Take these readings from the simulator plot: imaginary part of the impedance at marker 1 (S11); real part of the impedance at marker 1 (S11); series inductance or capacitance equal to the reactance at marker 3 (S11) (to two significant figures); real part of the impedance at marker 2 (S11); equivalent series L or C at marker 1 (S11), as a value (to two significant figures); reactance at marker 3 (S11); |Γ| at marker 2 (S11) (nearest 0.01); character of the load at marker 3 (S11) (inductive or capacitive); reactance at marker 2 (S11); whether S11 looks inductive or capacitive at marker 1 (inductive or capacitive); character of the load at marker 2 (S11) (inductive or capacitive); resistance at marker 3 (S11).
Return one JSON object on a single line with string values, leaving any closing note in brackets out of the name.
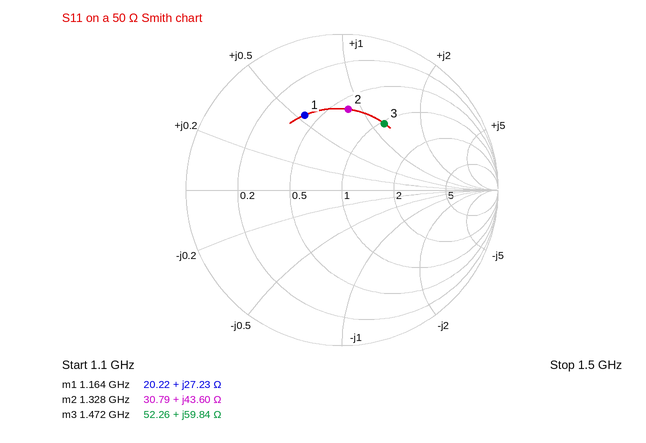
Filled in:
{"imaginary part of the impedance at marker 1": "+27.23 Ω", "real part of the impedance at marker 1": "20.22 Ω", "series inductance or capacitance equal to the reactance at marker 3 (S11)": "6.5 nH", "real part of the impedance at marker 2": "30.79 Ω", "equivalent series L or C at marker 1 (S11), as a value": "3.7 nH", "reactance at marker 3": "+59.84 Ω", "|Γ| at marker 2 (S11)": "0.52", "character of the load at marker 3 (S11)": "inductive", "reactance at marker 2": "+43.60 Ω", "whether S11 looks inductive or capacitive at marker 1": "inductive", "character of the load at marker 2 (S11)": "inductive", "resistance at marker 3": "52.26 Ω"}
